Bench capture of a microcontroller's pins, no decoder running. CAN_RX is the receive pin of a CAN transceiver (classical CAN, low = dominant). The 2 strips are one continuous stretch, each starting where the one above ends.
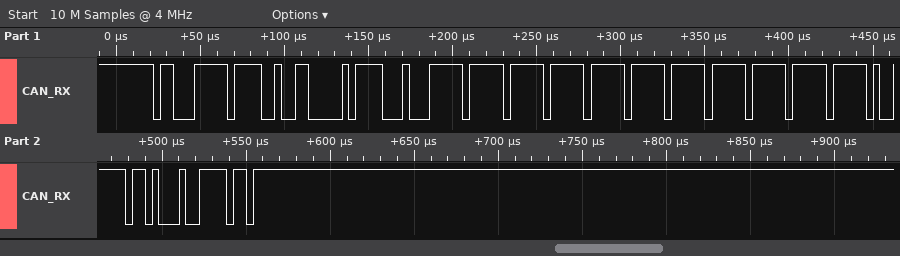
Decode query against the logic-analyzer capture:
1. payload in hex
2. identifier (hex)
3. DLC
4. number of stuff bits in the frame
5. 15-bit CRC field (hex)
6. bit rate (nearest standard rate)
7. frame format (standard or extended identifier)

FF FF FF FF FF FF FF 3D
0x18FE4C0F
8
13
0x513D
250 kbit/s
extended
